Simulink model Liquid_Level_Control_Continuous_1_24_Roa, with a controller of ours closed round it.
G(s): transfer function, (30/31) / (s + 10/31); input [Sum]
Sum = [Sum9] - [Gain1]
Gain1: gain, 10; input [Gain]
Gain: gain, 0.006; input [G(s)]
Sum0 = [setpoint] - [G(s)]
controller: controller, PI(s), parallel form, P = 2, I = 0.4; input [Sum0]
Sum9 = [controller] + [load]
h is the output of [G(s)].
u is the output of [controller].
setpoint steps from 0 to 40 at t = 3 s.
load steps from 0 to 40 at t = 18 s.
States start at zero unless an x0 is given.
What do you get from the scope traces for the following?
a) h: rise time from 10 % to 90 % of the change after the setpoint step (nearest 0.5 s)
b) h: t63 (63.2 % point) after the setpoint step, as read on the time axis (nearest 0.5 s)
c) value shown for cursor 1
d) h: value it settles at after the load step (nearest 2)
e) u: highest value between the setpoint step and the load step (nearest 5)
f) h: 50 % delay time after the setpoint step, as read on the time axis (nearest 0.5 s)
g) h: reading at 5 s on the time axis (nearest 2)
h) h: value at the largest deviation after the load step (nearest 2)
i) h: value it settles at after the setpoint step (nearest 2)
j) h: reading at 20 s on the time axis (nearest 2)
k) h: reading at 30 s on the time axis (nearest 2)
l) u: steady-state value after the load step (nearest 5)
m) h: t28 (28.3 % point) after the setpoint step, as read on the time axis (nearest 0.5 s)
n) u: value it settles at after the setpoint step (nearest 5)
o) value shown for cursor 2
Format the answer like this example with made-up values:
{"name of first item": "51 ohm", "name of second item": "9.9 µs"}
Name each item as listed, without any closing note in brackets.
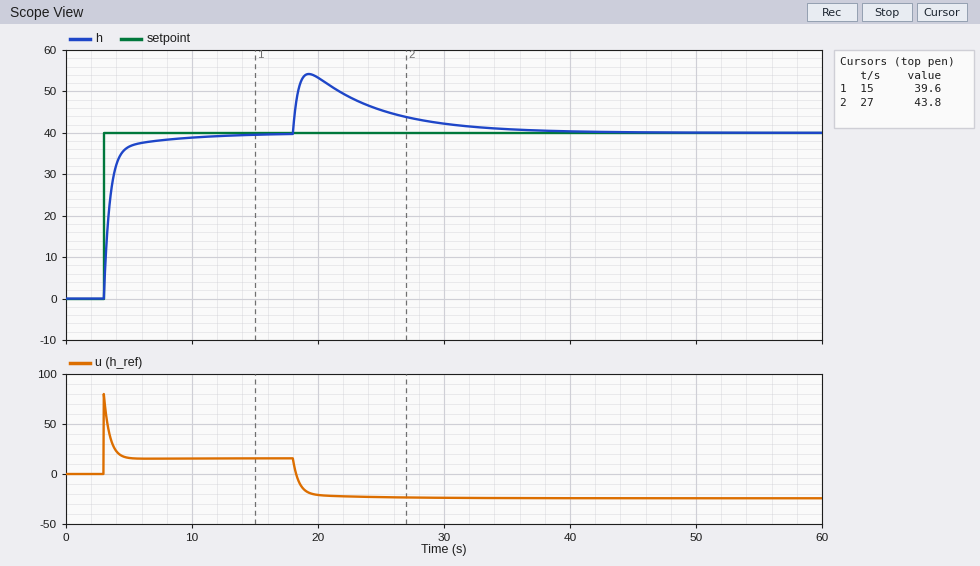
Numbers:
{"h: rise time from 10 % to 90 % of the change after the setpoint step": "1.5 s", "h: t63 (63.2 % point) after the setpoint step, as read on the time axis": "3.5 s", "value shown for cursor 1": "39.6", "h: value it settles at after the load step": "40", "u: highest value between the setpoint step and the load step": "80", "h: 50 % delay time after the setpoint step, as read on the time axis": "3.5 s", "h: reading at 5 s on the time axis": "36", "h: value at the largest deviation after the load step": "54", "h: value it settles at after the setpoint step": "40", "h: reading at 20 s on the time axis": "54", "h: reading at 30 s on the time axis": "42", "u: steady-state value after the load step": "-25", "h: t28 (28.3 % point) after the setpoint step, as read on the time axis": "3.0 s", "u: value it settles at after the setpoint step": "15", "value shown for cursor 2": "43.8"}
